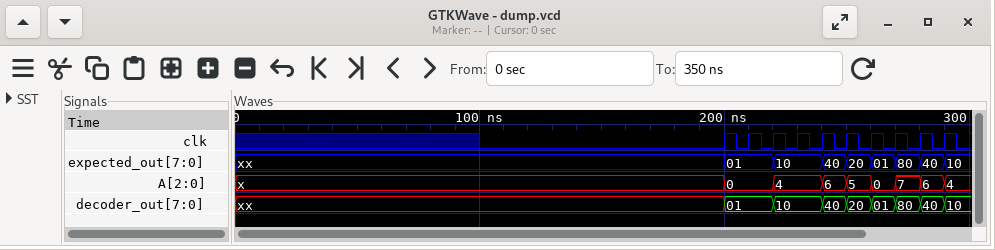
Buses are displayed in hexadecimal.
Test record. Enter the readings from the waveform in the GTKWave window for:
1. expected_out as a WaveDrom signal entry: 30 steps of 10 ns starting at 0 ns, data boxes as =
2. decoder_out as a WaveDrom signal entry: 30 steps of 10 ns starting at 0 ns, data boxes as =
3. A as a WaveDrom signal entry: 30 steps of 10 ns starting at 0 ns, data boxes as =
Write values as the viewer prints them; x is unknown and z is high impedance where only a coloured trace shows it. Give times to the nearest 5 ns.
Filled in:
{name: 'expected_out', wave: 'x...................=.=.======', data: '01 10 40 20 01 80 40 10'}
{name: 'decoder_out', wave: 'x...................=.=.======', data: '01 10 40 20 01 80 40 10'}
{name: 'A', wave: 'x...................=.=.======', data: '0 4 6 5 0 7 6 4'}
